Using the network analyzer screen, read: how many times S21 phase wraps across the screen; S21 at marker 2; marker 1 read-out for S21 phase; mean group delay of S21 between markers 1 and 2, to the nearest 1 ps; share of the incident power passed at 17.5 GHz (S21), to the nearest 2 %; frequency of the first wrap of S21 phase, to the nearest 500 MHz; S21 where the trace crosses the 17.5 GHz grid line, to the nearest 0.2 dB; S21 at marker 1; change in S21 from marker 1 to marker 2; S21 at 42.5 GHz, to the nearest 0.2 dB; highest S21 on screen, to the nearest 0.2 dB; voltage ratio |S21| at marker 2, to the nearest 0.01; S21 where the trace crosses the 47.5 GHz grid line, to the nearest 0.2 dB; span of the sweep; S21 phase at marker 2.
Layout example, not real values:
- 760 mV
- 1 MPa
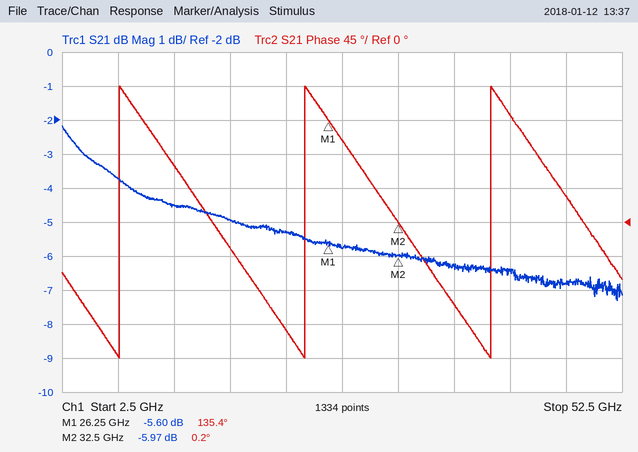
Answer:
- 3
- -5.97 dB
- 135.4°
- 60 ps
- 32 %
- 7.5 GHz
- -5.0 dB
- -5.60 dB
- -0.37 dB
- -6.4 dB
- -2.2 dB
- 0.50
- -6.8 dB
- 50 GHz
- 0.2°
